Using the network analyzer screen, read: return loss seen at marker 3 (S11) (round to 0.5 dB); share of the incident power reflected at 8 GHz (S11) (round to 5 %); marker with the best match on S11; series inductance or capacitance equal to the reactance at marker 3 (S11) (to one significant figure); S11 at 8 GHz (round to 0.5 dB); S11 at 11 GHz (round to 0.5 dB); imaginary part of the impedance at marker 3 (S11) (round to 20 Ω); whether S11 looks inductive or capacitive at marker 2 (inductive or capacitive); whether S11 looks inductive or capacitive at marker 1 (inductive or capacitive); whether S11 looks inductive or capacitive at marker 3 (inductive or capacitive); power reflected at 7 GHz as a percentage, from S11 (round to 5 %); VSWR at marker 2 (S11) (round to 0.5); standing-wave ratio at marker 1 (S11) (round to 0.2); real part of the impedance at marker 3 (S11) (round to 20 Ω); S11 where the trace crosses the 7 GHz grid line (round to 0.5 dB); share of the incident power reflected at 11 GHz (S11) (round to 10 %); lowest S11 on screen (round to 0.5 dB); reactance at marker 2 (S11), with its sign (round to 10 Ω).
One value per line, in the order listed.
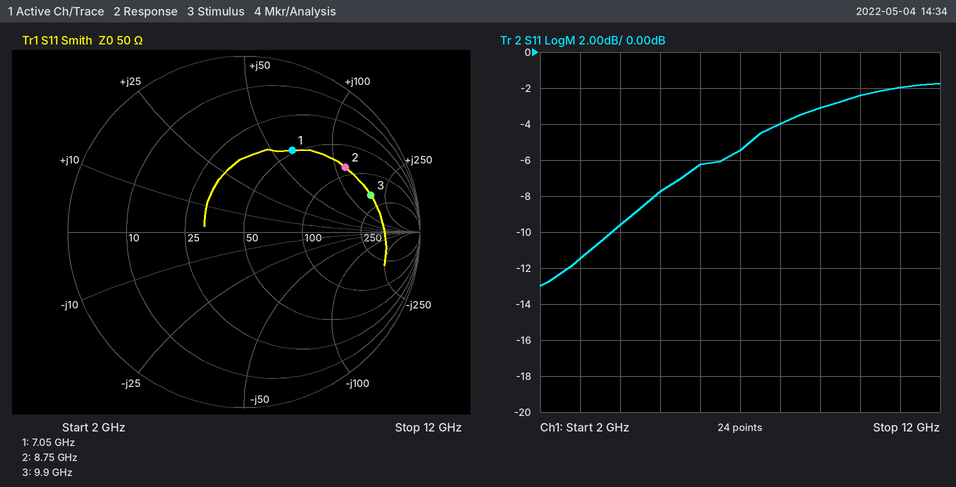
2.5 dB
40 %
marker 1
3 nH
-4.0 dB
-2.0 dB
+180 Ω
inductive
inductive
inductive
30 %
5.5
3.4
180 Ω
-5.5 dB
60 %
-13.0 dB
+120 Ω
